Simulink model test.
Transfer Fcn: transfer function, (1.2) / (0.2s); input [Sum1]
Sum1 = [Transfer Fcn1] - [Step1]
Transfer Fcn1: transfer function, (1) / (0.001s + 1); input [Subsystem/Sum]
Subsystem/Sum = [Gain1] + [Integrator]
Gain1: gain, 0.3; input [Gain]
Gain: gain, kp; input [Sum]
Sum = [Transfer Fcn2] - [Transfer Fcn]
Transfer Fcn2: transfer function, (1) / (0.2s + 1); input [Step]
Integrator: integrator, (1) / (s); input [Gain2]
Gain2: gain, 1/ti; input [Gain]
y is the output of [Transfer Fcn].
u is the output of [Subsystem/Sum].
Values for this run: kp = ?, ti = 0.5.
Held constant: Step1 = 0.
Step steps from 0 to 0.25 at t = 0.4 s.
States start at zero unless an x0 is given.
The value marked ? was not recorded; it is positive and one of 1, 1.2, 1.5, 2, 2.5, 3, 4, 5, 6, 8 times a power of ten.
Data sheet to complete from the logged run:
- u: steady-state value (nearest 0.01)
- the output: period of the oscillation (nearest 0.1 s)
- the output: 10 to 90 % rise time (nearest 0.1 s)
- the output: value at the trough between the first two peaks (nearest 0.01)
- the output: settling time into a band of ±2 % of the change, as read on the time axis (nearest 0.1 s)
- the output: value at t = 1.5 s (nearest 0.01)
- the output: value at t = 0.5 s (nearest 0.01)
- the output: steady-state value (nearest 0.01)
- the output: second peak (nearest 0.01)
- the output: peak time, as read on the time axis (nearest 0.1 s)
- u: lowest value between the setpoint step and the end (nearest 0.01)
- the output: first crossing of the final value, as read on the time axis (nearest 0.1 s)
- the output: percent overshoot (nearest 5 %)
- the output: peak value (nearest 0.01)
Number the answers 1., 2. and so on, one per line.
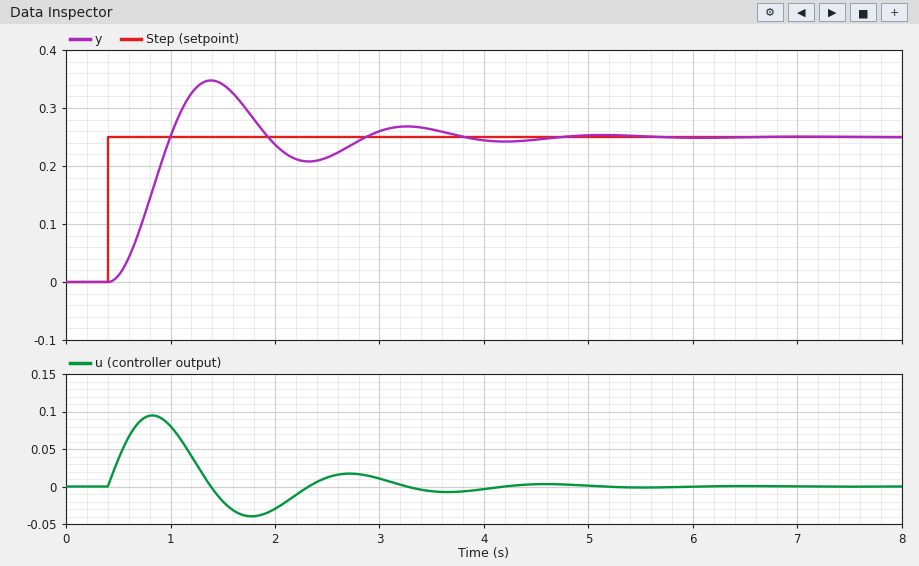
1. 0.00
2. 1.9 s
3. 0.4 s
4. 0.21
5. 4.5 s
6. 0.34
7. 0.01
8. 0.25
9. 0.27
10. 1.4 s
11. -0.04
12. 1.0 s
13. 40 %
14. 0.35
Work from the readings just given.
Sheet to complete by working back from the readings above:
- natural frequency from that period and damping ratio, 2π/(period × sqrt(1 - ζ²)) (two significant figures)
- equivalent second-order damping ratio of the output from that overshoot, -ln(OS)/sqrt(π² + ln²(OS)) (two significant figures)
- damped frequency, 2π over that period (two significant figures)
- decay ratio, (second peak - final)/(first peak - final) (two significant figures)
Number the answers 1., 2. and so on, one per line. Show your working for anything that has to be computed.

1. 2π / (1.9 × sqrt(1 - 0.28²)) = 3.4 rad/s
2. ln(0.4) = -0.916; 0.916 / sqrt(9.870 + 0.840) = 0.28
3. 2π / 1.9 = 3.3 rad/s
4. (0.27 - 0.25) / (0.35 - 0.25) = 0.20
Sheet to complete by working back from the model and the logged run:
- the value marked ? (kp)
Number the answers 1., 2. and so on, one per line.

1. 1
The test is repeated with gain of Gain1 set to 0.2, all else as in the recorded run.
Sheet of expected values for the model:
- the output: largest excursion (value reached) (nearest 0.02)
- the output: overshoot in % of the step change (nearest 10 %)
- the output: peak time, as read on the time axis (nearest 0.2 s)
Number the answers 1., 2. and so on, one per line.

1. 0.38
2. 50 %
3. 1.4 s
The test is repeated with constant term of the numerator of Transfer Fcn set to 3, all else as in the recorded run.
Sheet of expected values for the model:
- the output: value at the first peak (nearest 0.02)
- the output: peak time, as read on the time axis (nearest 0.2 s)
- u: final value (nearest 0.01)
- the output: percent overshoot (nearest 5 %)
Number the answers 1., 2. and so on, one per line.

1. 0.30
2. 1.0 s
3. 0.00
4. 20 %
